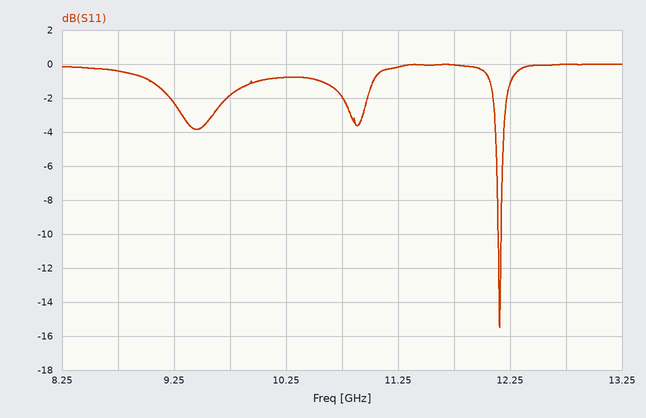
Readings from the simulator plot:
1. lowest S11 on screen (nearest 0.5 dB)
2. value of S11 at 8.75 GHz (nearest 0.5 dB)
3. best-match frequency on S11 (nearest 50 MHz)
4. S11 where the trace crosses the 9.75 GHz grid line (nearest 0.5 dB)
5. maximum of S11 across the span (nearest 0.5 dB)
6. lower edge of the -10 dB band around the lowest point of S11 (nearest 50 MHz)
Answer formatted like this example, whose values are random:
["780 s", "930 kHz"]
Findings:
["-15.5 dB", "-0.5 dB", "12.15 GHz", "-2.0 dB", "0.0 dB", "12.15 GHz"]
